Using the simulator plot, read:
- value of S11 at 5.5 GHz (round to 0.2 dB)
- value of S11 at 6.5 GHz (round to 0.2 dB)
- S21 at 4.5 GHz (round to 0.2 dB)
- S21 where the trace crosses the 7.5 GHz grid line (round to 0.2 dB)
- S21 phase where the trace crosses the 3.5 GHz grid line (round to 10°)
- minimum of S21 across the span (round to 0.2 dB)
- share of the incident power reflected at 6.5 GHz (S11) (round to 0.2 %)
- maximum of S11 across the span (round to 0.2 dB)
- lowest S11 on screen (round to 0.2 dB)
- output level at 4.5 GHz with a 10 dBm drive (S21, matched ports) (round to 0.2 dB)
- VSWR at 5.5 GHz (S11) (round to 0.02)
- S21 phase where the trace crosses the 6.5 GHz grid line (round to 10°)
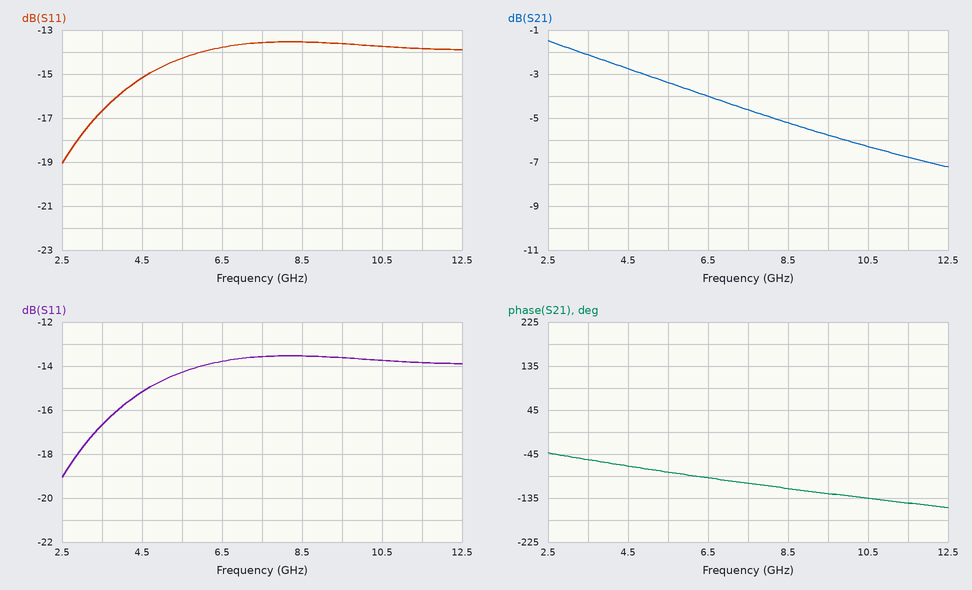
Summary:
-14.2 dB
-13.8 dB
-2.8 dB
-4.6 dB
-60°
-7.2 dB
4.2 %
-13.6 dB
-19.0 dB
7.2 dBm
1.48
-90°
